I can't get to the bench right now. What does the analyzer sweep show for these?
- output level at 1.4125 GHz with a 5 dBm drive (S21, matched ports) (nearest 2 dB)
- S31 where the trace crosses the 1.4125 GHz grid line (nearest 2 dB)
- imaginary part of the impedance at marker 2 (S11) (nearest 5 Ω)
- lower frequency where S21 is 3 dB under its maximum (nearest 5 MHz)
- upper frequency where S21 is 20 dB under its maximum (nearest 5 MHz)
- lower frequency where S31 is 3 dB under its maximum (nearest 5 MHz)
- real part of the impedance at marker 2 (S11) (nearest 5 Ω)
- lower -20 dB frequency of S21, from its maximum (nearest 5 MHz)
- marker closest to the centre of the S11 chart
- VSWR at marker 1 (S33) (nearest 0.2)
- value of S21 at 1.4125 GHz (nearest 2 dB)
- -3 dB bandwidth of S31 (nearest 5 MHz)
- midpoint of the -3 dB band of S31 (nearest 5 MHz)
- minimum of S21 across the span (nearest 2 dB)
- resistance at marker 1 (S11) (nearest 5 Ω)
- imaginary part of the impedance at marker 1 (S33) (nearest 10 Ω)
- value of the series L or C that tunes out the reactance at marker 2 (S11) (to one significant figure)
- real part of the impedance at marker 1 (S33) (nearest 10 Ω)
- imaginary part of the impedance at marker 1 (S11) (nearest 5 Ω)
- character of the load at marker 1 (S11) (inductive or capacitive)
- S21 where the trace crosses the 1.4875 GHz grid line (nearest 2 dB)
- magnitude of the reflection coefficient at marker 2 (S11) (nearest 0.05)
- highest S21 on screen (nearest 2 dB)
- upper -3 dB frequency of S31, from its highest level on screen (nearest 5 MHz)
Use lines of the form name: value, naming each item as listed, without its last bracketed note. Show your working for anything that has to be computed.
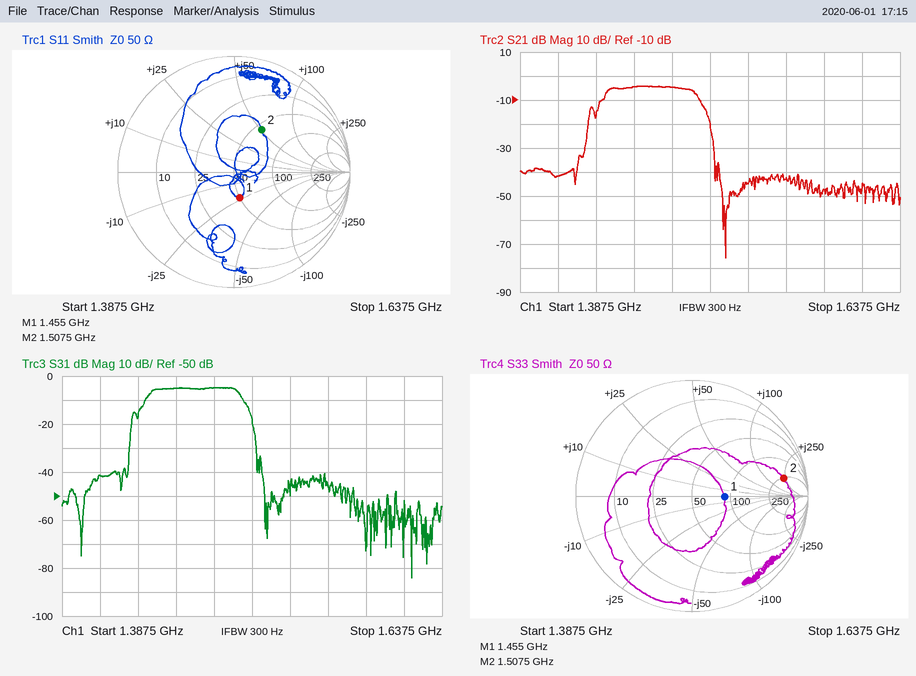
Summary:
output level at 1.4125 GHz with a 5 dBm drive (S21, matched ports): 5 dBm + (-42 dB) = -36 dBm
S31 where the trace crosses the 1.4125 GHz grid line: -42 dB
imaginary part of the impedance at marker 2 (S11): +50 Ω
lower frequency where S21 is 3 dB under its maximum: 1.445 GHz
upper frequency where S21 is 20 dB under its maximum: 1.515 GHz
lower frequency where S31 is 3 dB under its maximum: 1.445 GHz
real part of the impedance at marker 2 (S11): 55 Ω
lower -20 dB frequency of S21, from its maximum: 1.430 GHz
marker closest to the centre of the S11 chart: marker 1
VSWR at marker 1 (S33): 1.8
value of S21 at 1.4125 GHz: -42 dB
-3 dB bandwidth of S31: 1.505 GHz − 1.445 GHz = 60 MHz
midpoint of the -3 dB band of S31: 1.475 GHz
minimum of S21 across the span: -76 dB
resistance at marker 1 (S11): 50 Ω
imaginary part of the impedance at marker 1 (S33): 0 Ω
value of the series L or C that tunes out the reactance at marker 2 (S11): C = 1/(2π × 1.5075 GHz × 50 Ω) ≈ 2 pF
real part of the impedance at marker 1 (S33): 90 Ω
imaginary part of the impedance at marker 1 (S11): -25 Ω
character of the load at marker 1 (S11): capacitive
S21 where the trace crosses the 1.4875 GHz grid line: -4 dB
magnitude of the reflection coefficient at marker 2 (S11): 0.45
highest S21 on screen: -4 dB
upper -3 dB frequency of S31, from its highest level on screen: 1.505 GHz
